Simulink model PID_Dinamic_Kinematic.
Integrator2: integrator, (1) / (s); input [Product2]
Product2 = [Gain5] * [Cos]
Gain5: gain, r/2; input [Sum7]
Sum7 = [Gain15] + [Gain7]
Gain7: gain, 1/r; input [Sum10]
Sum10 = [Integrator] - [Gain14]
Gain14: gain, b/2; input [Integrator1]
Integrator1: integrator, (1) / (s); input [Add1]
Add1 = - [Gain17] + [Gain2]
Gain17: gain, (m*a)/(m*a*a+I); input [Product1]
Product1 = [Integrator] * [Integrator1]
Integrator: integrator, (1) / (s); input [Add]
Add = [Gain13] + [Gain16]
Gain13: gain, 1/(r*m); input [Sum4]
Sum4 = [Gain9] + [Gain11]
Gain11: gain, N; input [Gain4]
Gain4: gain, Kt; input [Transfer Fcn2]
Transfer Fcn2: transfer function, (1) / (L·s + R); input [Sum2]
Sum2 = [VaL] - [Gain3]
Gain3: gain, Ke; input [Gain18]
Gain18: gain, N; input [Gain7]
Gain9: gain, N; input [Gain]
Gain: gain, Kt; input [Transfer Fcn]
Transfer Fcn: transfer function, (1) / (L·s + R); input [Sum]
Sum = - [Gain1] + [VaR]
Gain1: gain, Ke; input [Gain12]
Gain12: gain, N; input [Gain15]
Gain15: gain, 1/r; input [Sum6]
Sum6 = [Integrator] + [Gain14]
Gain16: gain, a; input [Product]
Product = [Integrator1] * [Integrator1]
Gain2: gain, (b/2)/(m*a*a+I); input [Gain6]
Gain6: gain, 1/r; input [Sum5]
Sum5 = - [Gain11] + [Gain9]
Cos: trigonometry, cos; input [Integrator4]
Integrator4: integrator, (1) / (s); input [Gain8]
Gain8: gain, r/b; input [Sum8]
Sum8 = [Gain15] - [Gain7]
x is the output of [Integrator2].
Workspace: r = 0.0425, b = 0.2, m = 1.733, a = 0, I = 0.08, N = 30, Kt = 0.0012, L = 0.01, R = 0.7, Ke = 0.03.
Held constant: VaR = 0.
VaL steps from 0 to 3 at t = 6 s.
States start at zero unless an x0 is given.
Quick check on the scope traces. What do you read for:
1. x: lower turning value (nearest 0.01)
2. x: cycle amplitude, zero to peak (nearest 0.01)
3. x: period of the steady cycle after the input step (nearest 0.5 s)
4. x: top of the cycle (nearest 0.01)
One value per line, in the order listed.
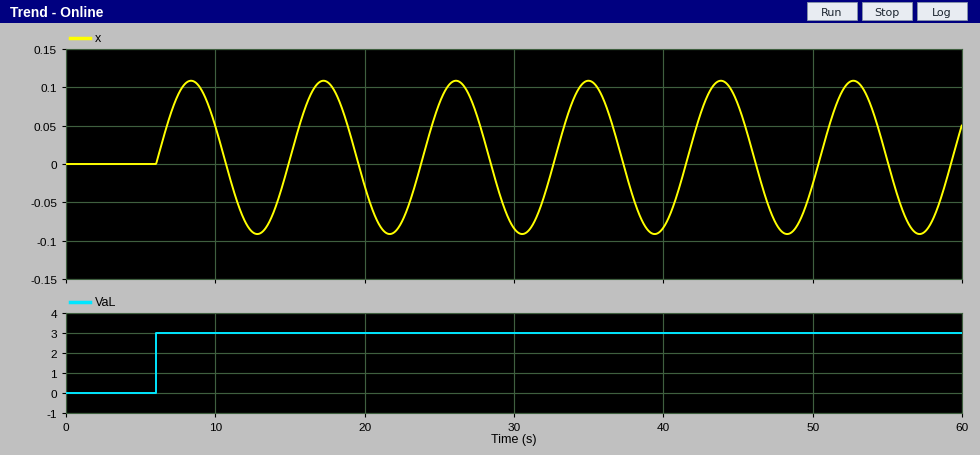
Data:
-0.09
0.10
9.0 s
0.11
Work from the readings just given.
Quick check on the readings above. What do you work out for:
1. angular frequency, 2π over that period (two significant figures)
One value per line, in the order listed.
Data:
0.70 rad/s
